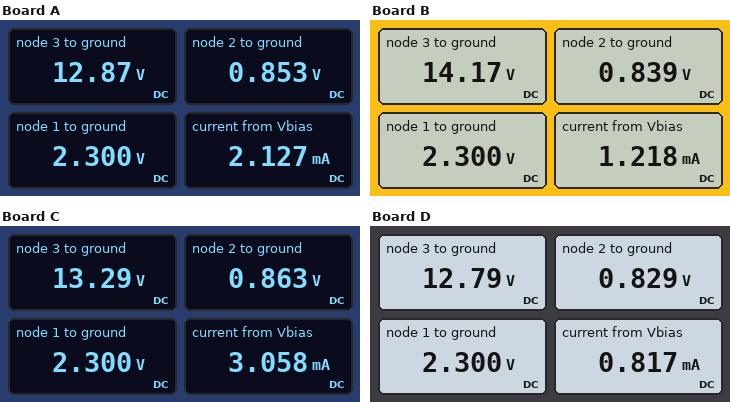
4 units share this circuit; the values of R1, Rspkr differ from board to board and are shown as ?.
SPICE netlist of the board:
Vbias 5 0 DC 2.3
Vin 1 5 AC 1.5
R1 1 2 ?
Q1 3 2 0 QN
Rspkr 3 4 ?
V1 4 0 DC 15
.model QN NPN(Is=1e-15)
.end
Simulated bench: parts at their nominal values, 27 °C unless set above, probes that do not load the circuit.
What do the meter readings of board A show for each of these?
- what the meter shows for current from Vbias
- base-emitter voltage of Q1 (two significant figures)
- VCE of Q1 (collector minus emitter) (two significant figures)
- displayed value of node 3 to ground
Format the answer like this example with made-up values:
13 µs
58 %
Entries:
2.127 mA
850 mV
13 V
12.87 V
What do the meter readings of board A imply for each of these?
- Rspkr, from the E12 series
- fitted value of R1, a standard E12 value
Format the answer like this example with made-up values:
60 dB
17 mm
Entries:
10 Ω
680 Ω
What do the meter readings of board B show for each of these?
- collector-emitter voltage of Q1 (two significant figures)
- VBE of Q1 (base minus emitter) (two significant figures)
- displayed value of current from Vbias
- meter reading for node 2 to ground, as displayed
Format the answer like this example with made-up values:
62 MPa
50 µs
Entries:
14 V
840 mV
1.218 mA
0.839 V
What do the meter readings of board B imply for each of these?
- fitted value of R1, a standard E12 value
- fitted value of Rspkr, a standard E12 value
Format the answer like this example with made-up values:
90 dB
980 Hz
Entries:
1.2 kΩ
6.8 Ω
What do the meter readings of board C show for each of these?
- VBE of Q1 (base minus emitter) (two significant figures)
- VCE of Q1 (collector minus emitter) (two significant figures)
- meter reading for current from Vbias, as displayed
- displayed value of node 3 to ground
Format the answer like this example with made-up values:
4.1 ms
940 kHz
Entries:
860 mV
13 V
3.058 mA
13.29 V
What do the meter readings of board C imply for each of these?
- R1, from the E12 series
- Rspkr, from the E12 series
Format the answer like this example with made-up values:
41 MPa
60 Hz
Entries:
470 Ω
5.6 Ω
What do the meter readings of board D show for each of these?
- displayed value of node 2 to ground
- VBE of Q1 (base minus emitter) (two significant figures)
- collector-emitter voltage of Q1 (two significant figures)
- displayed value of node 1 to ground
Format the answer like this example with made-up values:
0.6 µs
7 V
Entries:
0.829 V
830 mV
13 V
2.300 V
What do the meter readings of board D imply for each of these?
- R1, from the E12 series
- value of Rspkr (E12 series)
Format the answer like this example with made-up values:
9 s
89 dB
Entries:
1.8 kΩ
27 Ω
